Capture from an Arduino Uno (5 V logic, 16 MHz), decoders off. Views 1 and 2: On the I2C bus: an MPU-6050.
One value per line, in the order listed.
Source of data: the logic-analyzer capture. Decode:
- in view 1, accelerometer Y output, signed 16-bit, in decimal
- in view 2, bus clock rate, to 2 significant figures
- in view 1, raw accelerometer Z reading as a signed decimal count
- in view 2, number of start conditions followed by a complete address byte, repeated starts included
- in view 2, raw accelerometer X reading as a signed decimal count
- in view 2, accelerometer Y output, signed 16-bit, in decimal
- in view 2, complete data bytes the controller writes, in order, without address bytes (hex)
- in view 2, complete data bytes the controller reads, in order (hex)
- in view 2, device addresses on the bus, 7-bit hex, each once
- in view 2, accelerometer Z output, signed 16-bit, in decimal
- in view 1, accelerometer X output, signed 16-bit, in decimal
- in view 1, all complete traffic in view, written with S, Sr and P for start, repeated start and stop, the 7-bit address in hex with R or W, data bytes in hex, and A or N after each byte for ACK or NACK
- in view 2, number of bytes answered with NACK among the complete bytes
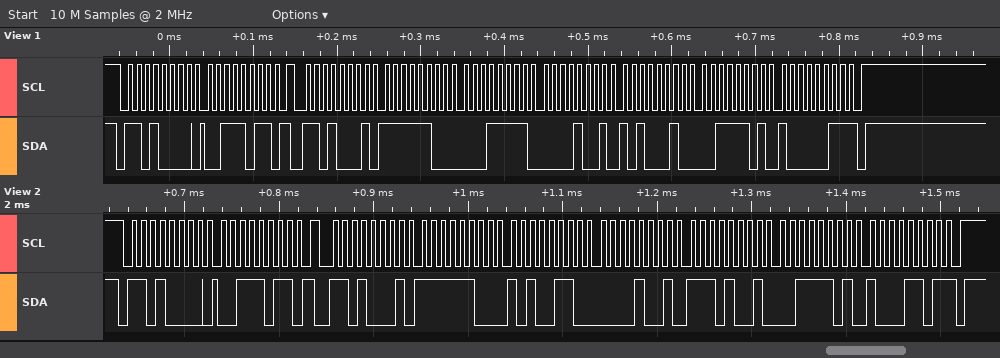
2466
100 kHz
15747
2
-858
2537
3B
FC A6 09 E9 3D 8D
0x68
15757
-993
S 68W A 3B A Sr 68R A FC A 1F A 09 A A2 A 3D A 83 N P
1
